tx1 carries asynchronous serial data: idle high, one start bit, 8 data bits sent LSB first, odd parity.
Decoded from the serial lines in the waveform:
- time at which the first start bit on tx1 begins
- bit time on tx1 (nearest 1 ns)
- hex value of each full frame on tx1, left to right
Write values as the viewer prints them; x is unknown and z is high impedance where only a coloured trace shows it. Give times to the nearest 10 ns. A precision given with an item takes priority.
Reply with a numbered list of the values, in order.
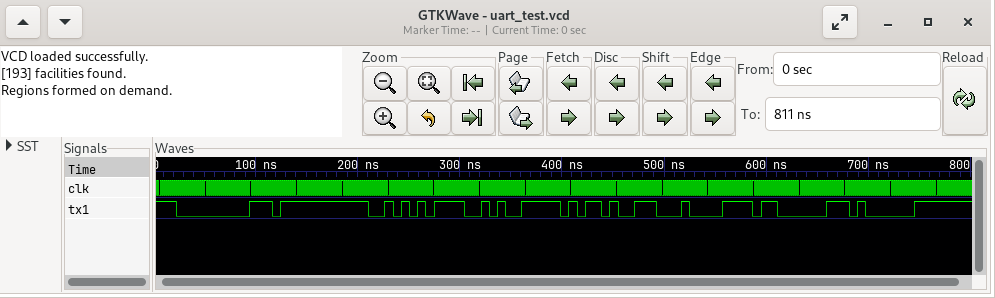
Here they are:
1. 20 ns
2. 8 ns
3. 00, FF, AA, CA, 2D, 84, 03, 81
